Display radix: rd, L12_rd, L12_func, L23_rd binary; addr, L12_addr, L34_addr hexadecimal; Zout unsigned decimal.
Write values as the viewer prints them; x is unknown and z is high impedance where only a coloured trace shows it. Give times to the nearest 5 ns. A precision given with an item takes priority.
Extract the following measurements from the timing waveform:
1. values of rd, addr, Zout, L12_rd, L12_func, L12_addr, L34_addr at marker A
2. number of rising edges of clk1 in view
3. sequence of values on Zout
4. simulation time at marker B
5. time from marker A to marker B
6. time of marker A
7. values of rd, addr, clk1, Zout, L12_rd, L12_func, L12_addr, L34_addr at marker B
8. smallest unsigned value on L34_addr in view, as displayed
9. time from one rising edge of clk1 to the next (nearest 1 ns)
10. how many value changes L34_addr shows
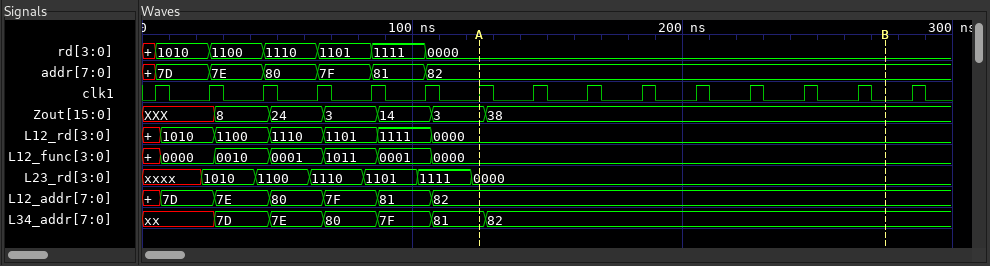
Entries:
rd=0000, addr=82, Zout=3, L12_rd=0000, L12_func=0000, L12_addr=82, L34_addr=81
15
XXX, 8, 24, 3, 14, 3, 38
275 ns
150 ns
125 ns
rd=0000, addr=82, clk1=0, Zout=38, L12_rd=0000, L12_func=0000, L12_addr=82, L34_addr=82
7D
20 ns
6
